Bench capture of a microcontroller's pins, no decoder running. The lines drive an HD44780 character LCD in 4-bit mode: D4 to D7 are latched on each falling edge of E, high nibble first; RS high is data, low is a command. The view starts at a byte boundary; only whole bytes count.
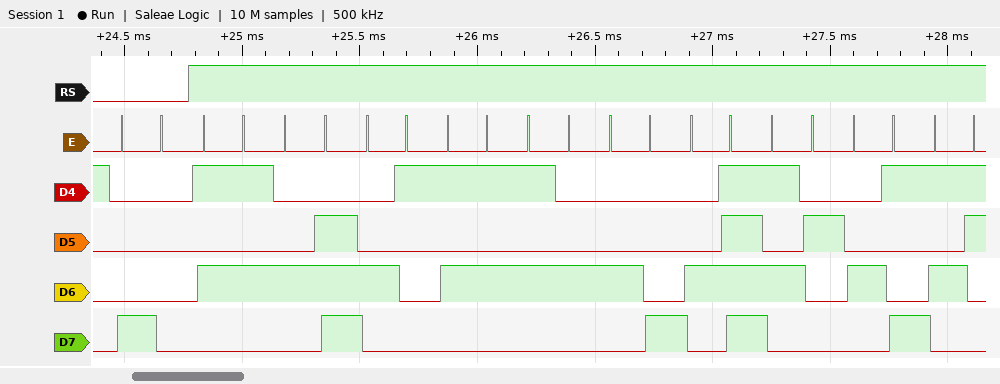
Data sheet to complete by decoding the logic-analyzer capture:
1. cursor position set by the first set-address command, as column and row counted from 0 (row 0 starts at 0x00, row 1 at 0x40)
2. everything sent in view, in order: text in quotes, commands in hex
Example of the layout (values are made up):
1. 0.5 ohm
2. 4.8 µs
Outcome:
1. column 0, row 0
2. 0x80 "UNAUTHORIS"
